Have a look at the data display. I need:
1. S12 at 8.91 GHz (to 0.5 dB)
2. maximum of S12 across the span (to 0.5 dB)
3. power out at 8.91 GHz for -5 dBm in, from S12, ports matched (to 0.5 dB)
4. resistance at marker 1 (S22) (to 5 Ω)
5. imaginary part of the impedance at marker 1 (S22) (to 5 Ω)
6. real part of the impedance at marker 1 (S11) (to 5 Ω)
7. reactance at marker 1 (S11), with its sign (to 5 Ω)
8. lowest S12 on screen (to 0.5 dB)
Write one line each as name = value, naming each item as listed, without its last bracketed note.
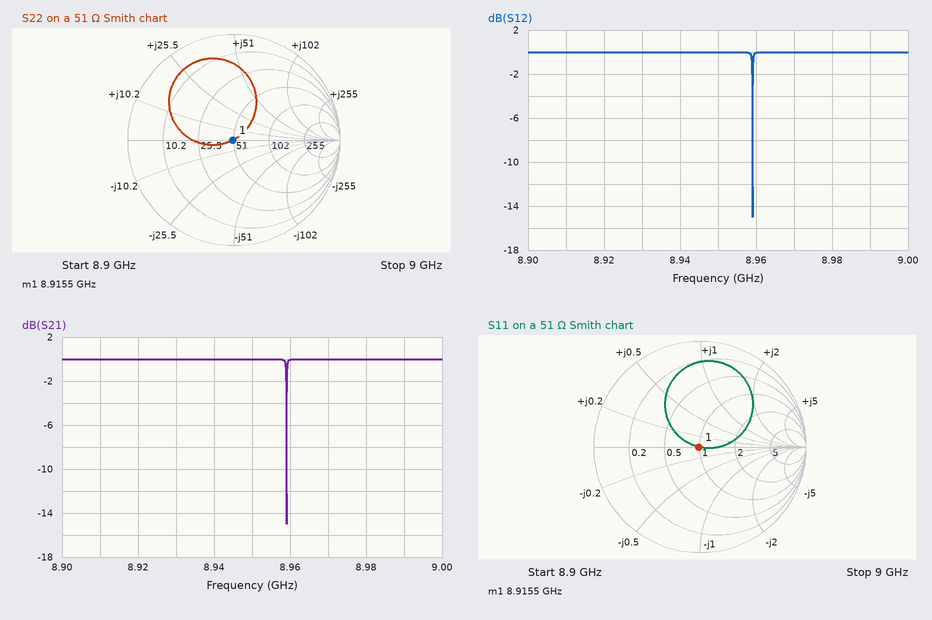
S12 at 8.91 GHz = 0.0 dB
maximum of S12 across the span = 0.0 dB
power out at 8.91 GHz for -5 dBm in, from S12, ports matched = -5.0 dBm
resistance at marker 1 (S22) = 50 Ω
imaginary part of the impedance at marker 1 (S22) = 0 Ω
real part of the impedance at marker 1 (S11) = 50 Ω
reactance at marker 1 (S11), with its sign = 0 Ω
lowest S12 on screen = -15.0 dB
